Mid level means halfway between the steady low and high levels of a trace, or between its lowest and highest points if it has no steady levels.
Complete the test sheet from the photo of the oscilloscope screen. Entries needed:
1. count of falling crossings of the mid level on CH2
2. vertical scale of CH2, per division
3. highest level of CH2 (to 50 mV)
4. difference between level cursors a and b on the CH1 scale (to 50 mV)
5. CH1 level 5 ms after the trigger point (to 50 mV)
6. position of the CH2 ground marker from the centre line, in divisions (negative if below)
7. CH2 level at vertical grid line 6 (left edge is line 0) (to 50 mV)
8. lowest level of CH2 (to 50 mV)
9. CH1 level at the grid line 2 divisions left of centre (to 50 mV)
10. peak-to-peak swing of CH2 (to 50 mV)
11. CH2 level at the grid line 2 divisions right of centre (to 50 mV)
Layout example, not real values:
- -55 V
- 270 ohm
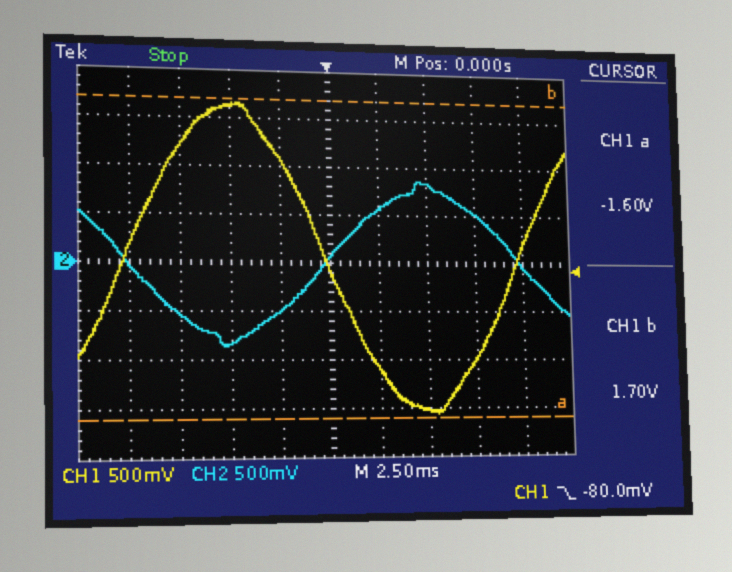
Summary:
- 2
- 500 mV
- 850 mV
- 3.30 V
- -1.50 V
- 0.0 div
- 550 mV
- -850 mV
- 1.65 V
- 1.70 V
- 850 mV
